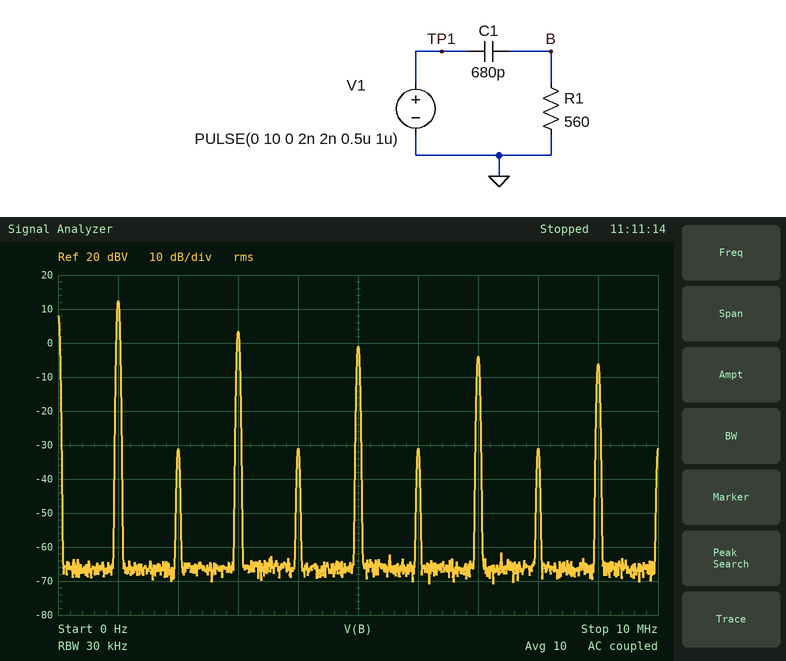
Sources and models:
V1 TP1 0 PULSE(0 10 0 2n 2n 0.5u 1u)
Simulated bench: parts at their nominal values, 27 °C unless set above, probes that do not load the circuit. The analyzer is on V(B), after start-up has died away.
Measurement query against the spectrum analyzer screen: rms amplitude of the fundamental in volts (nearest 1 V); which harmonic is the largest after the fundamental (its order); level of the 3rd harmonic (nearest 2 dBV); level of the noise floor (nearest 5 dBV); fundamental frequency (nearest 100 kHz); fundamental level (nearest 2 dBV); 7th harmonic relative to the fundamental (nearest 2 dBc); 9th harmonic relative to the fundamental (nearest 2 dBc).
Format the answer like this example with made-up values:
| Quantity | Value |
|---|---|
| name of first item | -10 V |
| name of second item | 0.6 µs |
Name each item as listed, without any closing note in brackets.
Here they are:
| Quantity | Value |
|---|---|
| rms amplitude of the fundamental in volts | 4 V |
| which harmonic is the largest after the fundamental | 3 |
| level of the 3rd harmonic | 4 dBV |
| level of the noise floor | -65 dBV |
| fundamental frequency | 1.0 MHz |
| fundamental level | 12 dBV |
| 7th harmonic relative to the fundamental | -16 dBc |
| 9th harmonic relative to the fundamental | -18 dBc |
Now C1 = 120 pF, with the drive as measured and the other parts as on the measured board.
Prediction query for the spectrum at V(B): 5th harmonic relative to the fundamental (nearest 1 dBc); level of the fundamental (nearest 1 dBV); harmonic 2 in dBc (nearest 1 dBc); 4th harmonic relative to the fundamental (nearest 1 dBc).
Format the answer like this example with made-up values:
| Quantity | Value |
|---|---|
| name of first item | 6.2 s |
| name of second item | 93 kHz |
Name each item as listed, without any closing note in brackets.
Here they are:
| Quantity | Value |
|---|---|
| 5th harmonic relative to the fundamental | -7 dBc |
| level of the fundamental | 5 dBV |
| harmonic 2 in dBc | -40 dBc |
| 4th harmonic relative to the fundamental | -37 dBc |
